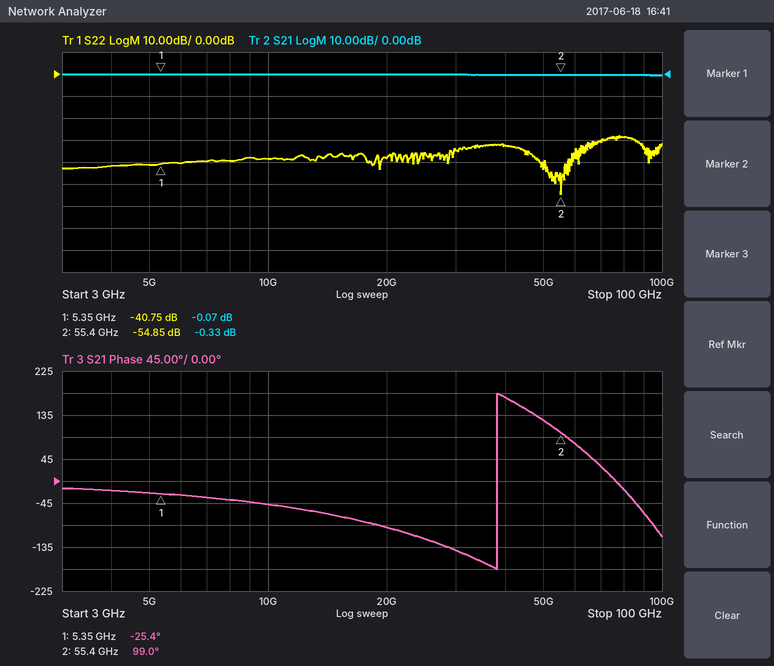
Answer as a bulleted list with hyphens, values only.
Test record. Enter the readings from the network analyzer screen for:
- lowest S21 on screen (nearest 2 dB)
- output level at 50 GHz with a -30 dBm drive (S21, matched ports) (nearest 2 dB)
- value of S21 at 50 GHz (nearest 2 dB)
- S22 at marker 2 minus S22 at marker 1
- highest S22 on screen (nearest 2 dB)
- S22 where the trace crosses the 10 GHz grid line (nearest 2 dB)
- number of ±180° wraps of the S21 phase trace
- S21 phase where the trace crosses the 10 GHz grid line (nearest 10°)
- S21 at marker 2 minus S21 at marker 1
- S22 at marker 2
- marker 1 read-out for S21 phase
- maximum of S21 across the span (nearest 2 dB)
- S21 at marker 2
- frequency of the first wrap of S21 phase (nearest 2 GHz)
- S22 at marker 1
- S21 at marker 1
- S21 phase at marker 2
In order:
- 0 dB
- -30 dBm
- 0 dB
- -14.10 dB
- -28 dB
- -38 dB
- 1
- -50°
- -0.26 dB
- -54.85 dB
- -25.4°
- 0 dB
- -0.33 dB
- 38 GHz
- -40.75 dB
- -0.07 dB
- 99.0°
